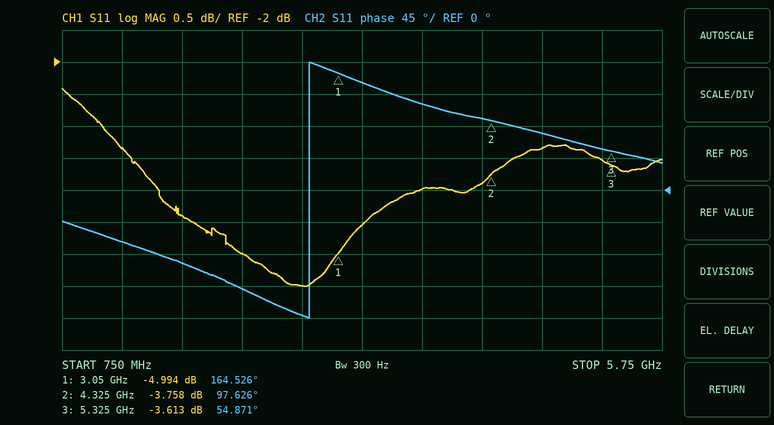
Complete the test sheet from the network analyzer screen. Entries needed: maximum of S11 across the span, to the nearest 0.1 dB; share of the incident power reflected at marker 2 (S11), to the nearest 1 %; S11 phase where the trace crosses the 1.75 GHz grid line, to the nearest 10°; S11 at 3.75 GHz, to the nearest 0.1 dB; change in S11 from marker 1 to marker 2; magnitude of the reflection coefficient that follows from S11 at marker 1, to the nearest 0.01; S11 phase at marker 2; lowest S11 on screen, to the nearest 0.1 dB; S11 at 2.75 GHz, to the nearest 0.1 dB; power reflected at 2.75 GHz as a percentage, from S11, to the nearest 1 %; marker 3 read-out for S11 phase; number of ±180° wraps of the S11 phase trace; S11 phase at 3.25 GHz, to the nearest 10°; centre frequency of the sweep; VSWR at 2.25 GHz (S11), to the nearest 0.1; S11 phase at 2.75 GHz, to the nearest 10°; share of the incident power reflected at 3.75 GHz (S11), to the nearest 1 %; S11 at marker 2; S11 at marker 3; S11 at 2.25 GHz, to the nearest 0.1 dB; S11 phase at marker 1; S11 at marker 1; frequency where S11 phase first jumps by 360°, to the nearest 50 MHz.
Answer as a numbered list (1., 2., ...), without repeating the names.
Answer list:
1. -2.4 dB
2. 42 %
3. -100°
4. -4.0 dB
5. 1.236 dB
6. 0.56
7. 97.626°
8. -5.5 dB
9. -5.5 dB
10. 28 %
11. 54.871°
12. 1
13. 150°
14. 3.25 GHz
15. 3.6
16. -180°
17. 40 %
18. -3.758 dB
19. -3.613 dB
20. -5.0 dB
21. 164.526°
22. -4.994 dB
23. 2.80 GHz
